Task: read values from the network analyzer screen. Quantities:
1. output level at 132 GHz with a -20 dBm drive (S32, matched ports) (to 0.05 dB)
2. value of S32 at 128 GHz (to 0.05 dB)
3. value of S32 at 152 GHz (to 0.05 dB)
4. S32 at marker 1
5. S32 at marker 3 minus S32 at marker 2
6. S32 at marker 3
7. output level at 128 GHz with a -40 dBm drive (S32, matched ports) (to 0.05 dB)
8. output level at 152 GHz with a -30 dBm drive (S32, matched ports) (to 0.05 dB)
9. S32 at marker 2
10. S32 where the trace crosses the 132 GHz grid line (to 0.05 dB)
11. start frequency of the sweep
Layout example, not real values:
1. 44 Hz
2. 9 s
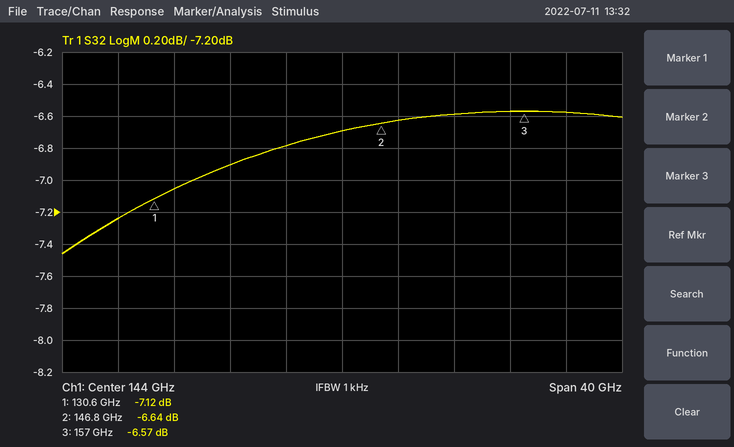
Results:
1. -27.05 dBm
2. -7.25 dB
3. -6.60 dB
4. -7.12 dB
5. 0.07 dB
6. -6.57 dB
7. -47.25 dBm
8. -36.60 dBm
9. -6.64 dB
10. -7.05 dB
11. 124 GHz
